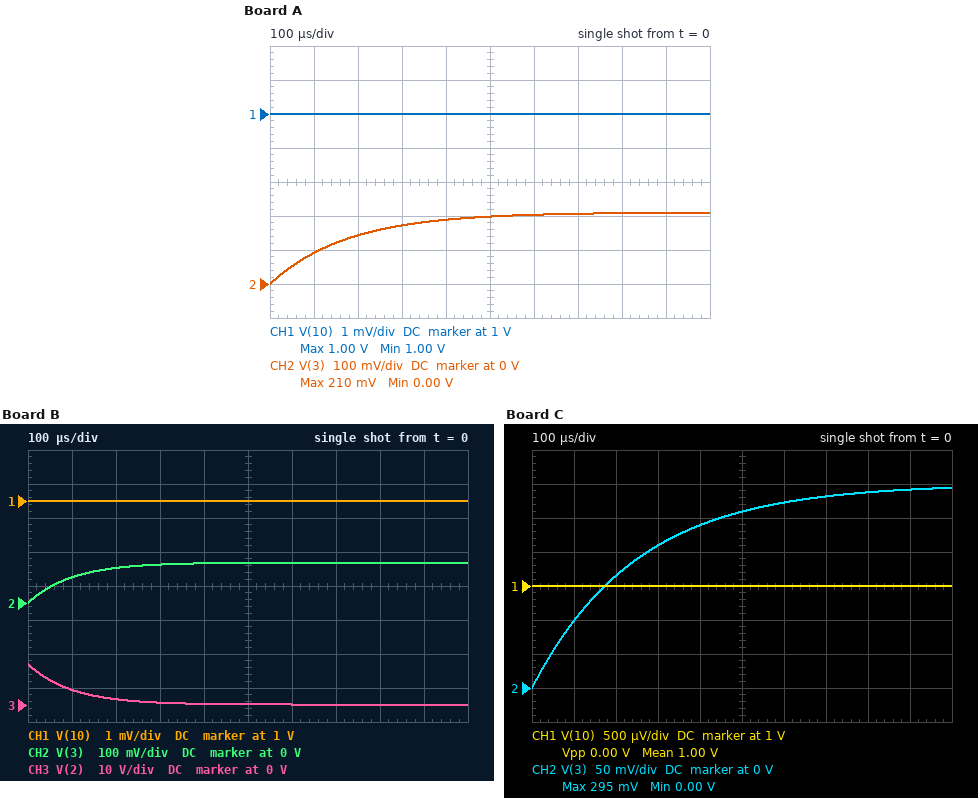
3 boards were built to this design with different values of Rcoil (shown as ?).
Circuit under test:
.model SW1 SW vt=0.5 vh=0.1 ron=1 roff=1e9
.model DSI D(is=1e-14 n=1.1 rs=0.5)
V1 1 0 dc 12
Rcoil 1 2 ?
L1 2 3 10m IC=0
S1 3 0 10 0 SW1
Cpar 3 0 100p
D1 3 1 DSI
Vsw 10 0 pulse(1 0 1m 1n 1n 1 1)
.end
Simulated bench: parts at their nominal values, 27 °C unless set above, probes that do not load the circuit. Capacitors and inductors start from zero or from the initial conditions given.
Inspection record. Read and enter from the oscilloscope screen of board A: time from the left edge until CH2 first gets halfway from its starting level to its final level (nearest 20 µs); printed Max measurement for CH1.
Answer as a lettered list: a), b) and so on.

a) 120 µs
b) 1.00 V
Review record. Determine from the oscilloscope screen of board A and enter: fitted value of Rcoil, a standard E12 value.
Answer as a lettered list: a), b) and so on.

a) 56 Ω
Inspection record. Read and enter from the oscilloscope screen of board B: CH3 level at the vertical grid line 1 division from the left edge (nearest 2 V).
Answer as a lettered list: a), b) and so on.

a) 4 V
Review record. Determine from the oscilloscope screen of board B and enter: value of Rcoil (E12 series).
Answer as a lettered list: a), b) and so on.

a) 100 Ω
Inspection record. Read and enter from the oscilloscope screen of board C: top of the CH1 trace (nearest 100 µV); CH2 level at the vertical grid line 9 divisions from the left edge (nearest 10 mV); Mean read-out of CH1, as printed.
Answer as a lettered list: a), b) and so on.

a) 1.0000 V
b) 290 mV
c) 1.00 V
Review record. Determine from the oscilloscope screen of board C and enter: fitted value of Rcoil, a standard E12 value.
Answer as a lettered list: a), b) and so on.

a) 39 Ω
